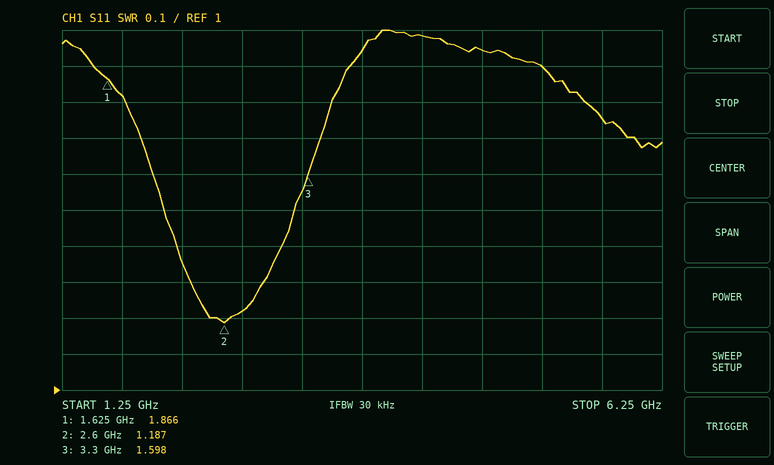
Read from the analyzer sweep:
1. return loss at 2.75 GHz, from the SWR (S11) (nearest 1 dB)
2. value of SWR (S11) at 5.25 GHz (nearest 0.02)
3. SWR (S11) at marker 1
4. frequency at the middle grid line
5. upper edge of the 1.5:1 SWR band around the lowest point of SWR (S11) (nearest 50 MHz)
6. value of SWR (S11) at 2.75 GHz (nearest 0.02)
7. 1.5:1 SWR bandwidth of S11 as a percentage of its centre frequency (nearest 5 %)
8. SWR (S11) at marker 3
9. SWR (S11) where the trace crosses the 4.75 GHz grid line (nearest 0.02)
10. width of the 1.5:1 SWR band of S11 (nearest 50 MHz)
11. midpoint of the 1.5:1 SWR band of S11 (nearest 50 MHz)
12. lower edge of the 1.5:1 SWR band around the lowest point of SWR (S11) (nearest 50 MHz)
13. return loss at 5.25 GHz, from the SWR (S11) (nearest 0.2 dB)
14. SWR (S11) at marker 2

20 dB
1.90
1.866
3.75 GHz
3.20 GHz
1.22
40 %
1.598
1.94
1.10 GHz
2.65 GHz
2.10 GHz
10.2 dB
1.187
